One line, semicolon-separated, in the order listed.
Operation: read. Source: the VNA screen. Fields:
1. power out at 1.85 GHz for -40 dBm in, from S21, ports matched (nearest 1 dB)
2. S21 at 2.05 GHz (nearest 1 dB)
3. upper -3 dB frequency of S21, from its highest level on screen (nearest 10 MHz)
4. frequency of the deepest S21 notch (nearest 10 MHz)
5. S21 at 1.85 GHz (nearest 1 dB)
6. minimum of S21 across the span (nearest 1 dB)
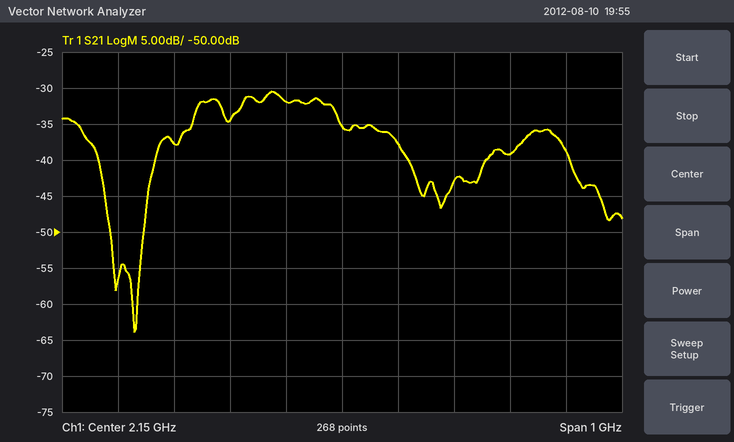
-78 dBm; -32 dB; 2.14 GHz; 1.78 GHz; -38 dB; -64 dB
